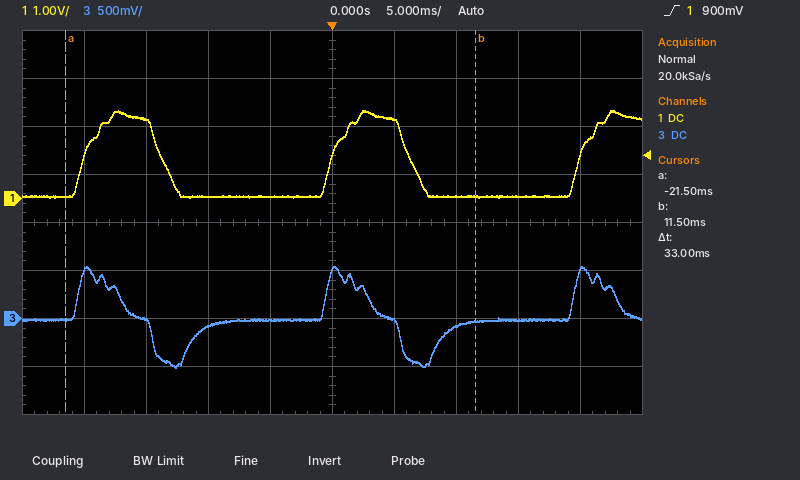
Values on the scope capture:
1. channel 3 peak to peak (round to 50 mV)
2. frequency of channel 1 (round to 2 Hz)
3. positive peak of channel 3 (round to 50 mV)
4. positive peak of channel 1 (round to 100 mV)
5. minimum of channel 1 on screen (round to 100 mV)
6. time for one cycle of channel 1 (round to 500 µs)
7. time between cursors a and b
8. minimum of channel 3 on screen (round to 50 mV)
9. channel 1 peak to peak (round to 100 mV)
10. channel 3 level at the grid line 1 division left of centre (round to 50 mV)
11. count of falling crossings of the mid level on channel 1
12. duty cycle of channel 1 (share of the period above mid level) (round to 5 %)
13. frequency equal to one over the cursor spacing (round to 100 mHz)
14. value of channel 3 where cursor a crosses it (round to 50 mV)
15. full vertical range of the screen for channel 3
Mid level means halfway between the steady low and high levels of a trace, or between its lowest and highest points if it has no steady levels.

1.05 V
50 Hz
550 mV
1.8 V
0.0 V
20.0 ms
33 ms
-500 mV
1.8 V
0 mV
2
30 %
30.3 Hz
0 mV
4 V
